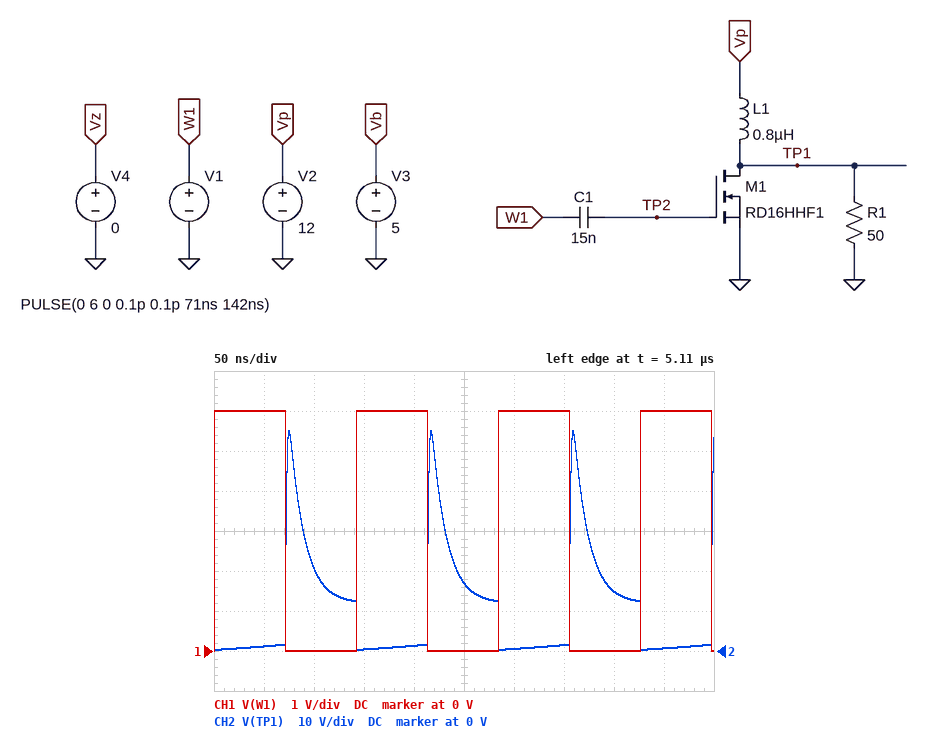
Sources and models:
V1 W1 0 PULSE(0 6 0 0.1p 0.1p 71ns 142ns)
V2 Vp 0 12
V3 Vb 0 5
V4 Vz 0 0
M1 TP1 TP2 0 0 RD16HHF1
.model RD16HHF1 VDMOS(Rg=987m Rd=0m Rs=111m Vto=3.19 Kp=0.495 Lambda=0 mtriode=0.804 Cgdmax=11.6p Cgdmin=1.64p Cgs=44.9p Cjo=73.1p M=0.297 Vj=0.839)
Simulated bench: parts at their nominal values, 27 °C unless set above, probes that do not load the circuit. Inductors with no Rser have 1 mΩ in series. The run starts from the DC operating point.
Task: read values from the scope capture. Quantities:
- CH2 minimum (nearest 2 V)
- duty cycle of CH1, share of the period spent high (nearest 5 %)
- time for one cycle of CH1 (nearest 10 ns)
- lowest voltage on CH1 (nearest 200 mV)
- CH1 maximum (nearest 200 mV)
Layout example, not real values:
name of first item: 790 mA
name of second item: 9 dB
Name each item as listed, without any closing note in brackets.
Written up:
CH2 minimum: 0 V
duty cycle of CH1, share of the period spent high: 50 %
time for one cycle of CH1: 140 ns
lowest voltage on CH1: 0 V
CH1 maximum: 6.0 V
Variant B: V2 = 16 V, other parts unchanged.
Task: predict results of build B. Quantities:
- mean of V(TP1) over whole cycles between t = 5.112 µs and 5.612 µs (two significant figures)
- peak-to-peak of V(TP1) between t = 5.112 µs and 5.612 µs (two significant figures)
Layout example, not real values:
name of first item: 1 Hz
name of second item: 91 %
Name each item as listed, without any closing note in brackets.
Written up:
mean of V(TP1) over whole cycles between t = 5.112 µs and 5.612 µs: 16 V
peak-to-peak of V(TP1) between t = 5.112 µs and 5.612 µs: 73 V
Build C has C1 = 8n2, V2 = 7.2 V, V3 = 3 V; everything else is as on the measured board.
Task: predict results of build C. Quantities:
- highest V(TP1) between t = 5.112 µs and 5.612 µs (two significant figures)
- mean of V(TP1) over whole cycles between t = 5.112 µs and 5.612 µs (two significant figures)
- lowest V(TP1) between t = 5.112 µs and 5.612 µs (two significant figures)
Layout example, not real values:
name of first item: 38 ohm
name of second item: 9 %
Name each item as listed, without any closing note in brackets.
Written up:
highest V(TP1) between t = 5.112 µs and 5.612 µs: 33 V
mean of V(TP1) over whole cycles between t = 5.112 µs and 5.612 µs: 7.2 V
lowest V(TP1) between t = 5.112 µs and 5.612 µs: 160 mV
